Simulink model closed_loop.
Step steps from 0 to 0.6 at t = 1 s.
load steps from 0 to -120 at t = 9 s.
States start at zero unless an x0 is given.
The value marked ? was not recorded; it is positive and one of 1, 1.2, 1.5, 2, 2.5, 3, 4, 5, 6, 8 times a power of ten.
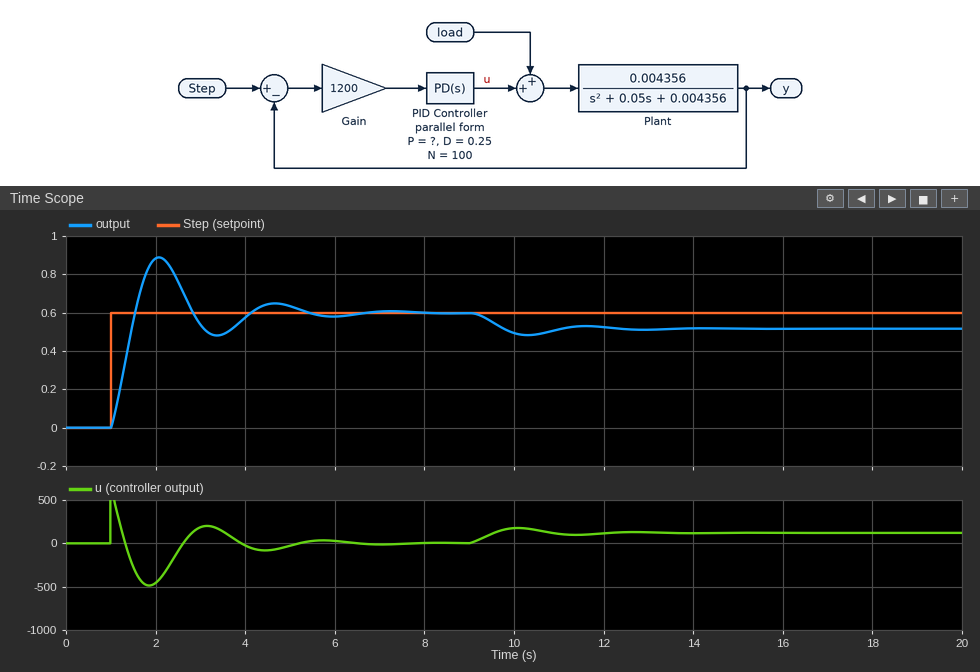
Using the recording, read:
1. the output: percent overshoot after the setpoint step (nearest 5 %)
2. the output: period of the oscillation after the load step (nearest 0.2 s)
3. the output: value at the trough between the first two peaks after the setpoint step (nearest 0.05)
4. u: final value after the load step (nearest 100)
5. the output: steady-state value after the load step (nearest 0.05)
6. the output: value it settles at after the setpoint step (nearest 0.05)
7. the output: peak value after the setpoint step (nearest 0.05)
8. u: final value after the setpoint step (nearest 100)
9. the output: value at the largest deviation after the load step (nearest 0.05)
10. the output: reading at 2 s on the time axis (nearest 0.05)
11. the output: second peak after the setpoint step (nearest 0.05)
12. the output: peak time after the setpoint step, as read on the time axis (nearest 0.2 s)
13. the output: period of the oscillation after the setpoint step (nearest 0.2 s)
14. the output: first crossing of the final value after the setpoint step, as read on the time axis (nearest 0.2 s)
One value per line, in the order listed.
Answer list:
50 %
2.6 s
0.50
100
0.50
0.60
0.90
0
0.50
0.90
0.65
2.0 s
2.6 s
1.6 s
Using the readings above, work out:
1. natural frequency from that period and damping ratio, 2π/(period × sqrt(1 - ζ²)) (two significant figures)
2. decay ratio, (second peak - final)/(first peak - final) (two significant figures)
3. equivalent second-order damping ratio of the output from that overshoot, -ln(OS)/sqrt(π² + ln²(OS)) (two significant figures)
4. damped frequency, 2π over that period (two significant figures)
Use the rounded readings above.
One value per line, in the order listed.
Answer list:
2.5 rad/s
0.17
0.22
2.4 rad/s
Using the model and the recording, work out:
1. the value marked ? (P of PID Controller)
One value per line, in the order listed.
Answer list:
1.2
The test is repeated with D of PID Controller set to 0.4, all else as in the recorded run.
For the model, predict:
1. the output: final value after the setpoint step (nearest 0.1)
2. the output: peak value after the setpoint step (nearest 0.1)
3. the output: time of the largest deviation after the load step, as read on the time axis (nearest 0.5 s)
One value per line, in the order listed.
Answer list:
0.6
0.8
10.5 s
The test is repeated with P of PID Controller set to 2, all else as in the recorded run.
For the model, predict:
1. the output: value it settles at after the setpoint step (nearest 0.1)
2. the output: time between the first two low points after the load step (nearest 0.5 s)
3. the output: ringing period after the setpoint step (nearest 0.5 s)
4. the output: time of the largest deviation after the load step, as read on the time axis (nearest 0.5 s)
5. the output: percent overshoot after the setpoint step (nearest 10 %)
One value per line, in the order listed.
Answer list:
0.6
2.0 s
2.0 s
10.0 s
60 %
